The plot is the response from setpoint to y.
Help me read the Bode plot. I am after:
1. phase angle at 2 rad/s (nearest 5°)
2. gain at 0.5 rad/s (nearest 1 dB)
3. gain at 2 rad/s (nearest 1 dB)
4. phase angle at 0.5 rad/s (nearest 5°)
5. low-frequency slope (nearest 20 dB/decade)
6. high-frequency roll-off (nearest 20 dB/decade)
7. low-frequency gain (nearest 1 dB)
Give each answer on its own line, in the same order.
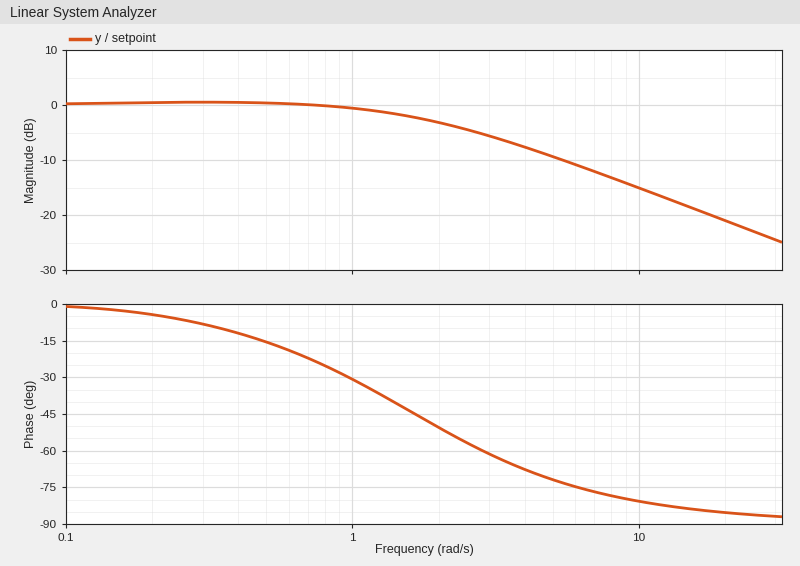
-50°
0 dB
-3 dB
-15°
0 dB/decade
-20 dB/decade
0 dB
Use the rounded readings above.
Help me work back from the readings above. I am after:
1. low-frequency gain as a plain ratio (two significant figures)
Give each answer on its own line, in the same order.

1.0
